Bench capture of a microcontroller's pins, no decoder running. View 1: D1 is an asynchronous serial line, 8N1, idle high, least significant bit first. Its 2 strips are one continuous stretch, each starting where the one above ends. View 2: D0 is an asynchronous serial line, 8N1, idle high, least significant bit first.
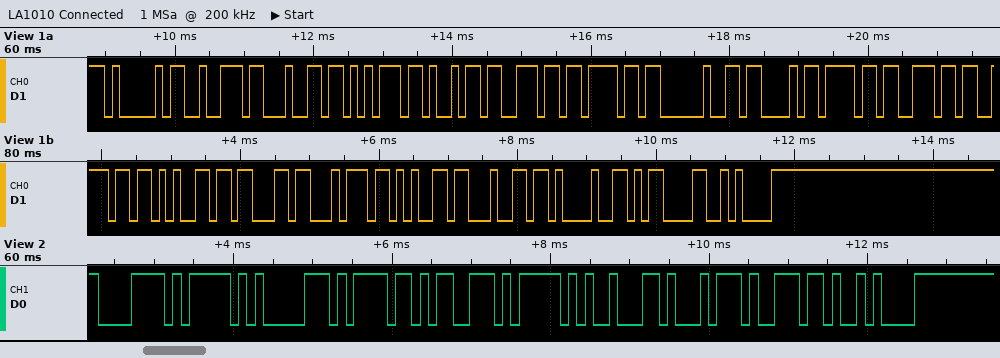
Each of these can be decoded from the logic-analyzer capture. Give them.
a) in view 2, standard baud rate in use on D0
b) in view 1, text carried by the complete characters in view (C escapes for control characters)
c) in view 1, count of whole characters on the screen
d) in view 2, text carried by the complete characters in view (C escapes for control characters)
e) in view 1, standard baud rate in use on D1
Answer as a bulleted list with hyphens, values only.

- 9600 baud
- "Arduino Connected!\r\n"
- 20
- "x_pos_btn\n"
- 9600 baud
